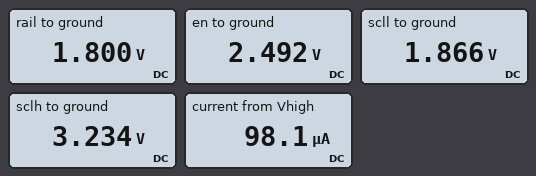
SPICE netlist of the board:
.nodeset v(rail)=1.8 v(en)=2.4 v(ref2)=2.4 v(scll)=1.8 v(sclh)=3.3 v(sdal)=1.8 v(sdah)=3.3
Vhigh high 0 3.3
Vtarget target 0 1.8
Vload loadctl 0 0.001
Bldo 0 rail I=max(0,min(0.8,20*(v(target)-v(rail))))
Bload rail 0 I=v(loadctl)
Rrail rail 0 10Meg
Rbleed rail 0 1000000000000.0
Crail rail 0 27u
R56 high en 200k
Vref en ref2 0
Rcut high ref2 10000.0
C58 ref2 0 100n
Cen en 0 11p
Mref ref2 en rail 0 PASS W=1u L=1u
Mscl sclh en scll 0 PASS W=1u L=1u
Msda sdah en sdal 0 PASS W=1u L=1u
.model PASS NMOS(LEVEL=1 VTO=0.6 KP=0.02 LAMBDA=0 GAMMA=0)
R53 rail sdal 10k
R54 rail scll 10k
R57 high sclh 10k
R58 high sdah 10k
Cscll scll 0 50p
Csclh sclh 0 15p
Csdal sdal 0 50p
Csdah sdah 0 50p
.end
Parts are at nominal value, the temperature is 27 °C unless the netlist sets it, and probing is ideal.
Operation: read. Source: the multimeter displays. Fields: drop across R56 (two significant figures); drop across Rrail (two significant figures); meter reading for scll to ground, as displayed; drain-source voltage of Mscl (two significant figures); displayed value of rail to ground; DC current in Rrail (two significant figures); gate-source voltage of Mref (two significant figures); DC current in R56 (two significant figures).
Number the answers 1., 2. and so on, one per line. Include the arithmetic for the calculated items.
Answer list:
1. 3.3 V - 2.492 V = 810 mV
2. 1.8 V = 1.8 V
3. 1.866 V
4. 3.234 V - 1.866 V = 1.4 V
5. 1.800 V
6. (1.8 V) / 10 MΩ = 180 nA
7. 2.492 V - 1.8 V = 690 mV
8. (3.3 V - 2.492 V) / 200 kΩ = 4.0 µA
